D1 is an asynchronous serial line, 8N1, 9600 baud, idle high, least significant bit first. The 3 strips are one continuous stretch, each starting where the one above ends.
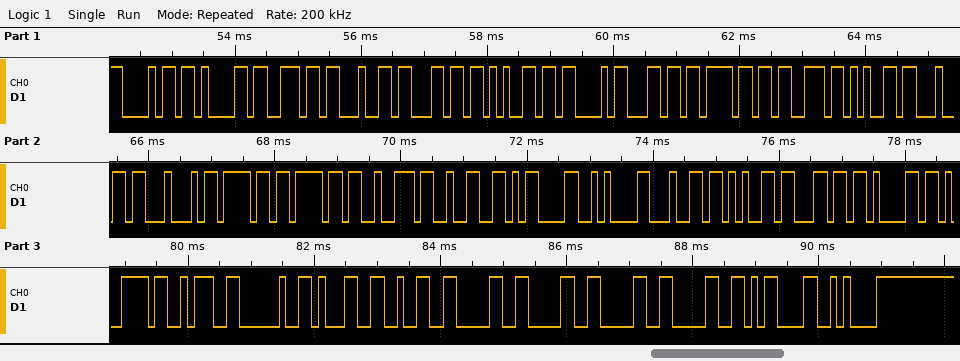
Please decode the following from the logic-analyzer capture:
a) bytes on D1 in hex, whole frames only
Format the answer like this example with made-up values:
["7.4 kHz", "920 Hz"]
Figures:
["68 61 6E 64 6C 65 43 6C 6F 73 65 64 44 6F 6F 72 32 0D 0A 64 65 6C 61 79 3A 20 31 32 30 30 30 30 0D 0A"]
